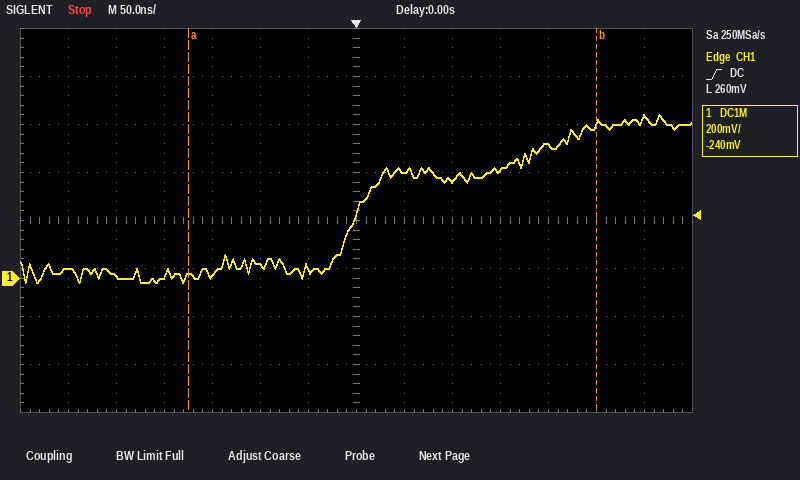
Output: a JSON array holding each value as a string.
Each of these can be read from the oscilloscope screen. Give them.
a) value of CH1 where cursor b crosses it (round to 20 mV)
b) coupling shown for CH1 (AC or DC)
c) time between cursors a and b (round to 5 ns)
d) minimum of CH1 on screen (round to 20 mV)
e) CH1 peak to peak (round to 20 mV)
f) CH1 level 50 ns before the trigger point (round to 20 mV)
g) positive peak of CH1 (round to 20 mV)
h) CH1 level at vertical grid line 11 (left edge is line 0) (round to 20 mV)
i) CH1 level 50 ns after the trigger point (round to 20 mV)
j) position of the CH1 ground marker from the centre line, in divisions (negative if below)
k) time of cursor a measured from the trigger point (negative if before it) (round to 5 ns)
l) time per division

["640 mV", "DC", "425 ns", "-20 mV", "700 mV", "40 mV", "680 mV", "560 mV", "440 mV", "-1.2 div", "-175 ns", "50 ns"]
